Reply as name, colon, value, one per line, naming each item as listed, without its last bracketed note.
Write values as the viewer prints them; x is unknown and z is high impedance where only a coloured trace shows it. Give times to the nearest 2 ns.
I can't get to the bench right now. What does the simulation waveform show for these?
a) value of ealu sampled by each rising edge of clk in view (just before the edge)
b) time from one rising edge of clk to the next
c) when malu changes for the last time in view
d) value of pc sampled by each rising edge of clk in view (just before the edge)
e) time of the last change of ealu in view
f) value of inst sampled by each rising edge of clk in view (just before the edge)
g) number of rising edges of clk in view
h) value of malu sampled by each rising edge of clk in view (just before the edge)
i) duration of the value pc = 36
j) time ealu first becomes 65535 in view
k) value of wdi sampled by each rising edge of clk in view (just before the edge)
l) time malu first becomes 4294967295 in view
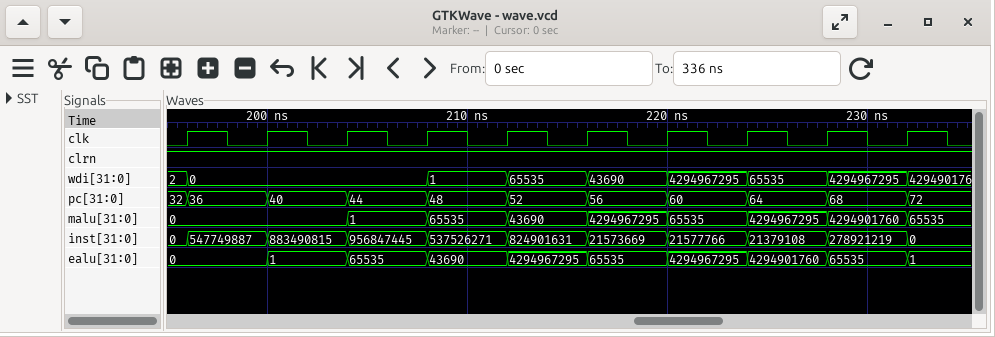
value of ealu sampled by each rising edge of clk in view: 0, 0, 1, 65535, 43690, 4294967295, 65535, 4294967295, 4294901760, 65535
time from one rising edge of clk to the next: 4 ns
when malu changes for the last time in view: 232 ns
value of pc sampled by each rising edge of clk in view: 32, 36, 40, 44, 48, 52, 56, 60, 64, 68
time of the last change of ealu in view: 232 ns
value of inst sampled by each rising edge of clk in view: 0, 547749887, 883490815, 956847445, 537526271, 824901631, 21573669, 21577766, 21379108, 278921219
number of rising edges of clk in view: 10
value of malu sampled by each rising edge of clk in view: 0, 0, 0, 1, 65535, 43690, 4294967295, 65535, 4294967295, 4294901760
duration of the value pc = 36: 4 ns
time ealu first becomes 65535 in view: 204 ns
value of wdi sampled by each rising edge of clk in view: 2, 0, 0, 0, 1, 65535, 43690, 4294967295, 65535, 4294967295
time malu first becomes 4294967295 in view: 216 ns
